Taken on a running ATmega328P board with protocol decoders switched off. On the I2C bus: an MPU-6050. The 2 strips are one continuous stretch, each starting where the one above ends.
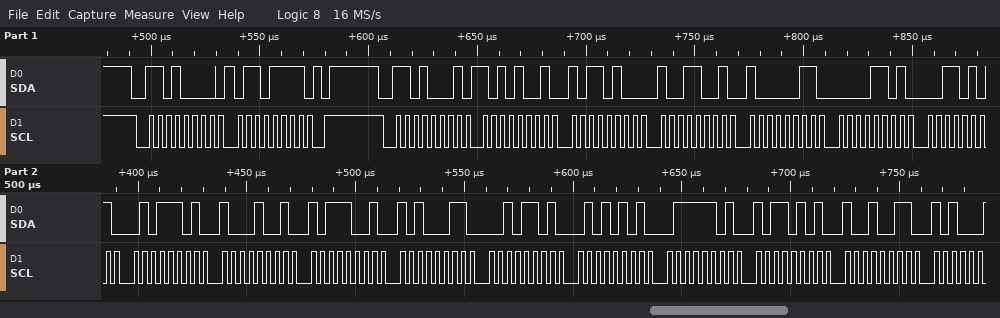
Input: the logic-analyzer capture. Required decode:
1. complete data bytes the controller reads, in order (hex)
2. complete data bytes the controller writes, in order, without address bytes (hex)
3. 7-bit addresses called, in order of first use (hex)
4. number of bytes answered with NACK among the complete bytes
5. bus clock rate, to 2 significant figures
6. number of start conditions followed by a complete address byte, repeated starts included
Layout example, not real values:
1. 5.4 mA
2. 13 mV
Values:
1. A9 B4 99 83 0D 35 5D 89 B9 A3 2D 55 7D B5 93
2. 6F
3. 0x68
4. 0
5. 250 kHz
6. 2
